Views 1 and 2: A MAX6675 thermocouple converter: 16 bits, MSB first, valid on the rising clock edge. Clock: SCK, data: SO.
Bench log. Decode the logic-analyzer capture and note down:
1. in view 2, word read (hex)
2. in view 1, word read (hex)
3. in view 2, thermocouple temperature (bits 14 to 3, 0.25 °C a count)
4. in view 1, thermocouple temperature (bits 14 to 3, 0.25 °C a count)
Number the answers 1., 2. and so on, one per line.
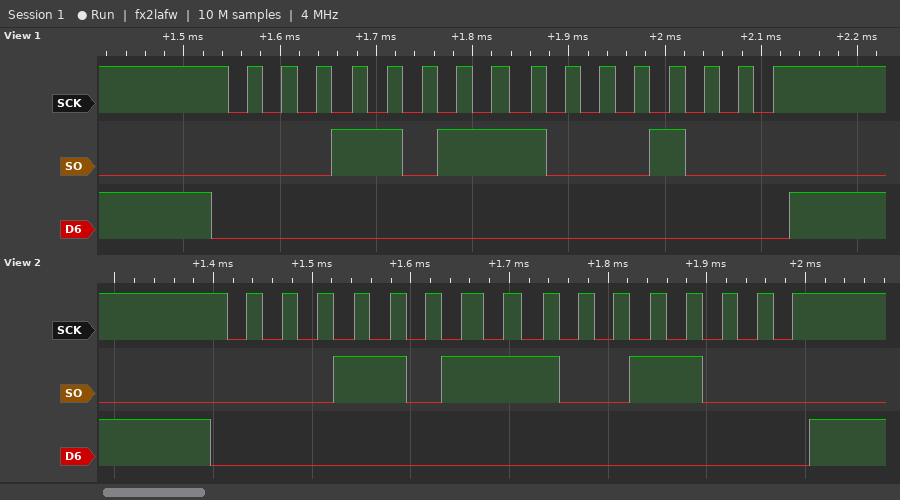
1. 0x1B98
2. 0x1B88
3. 220.75 °C
4. 220.25 °C
